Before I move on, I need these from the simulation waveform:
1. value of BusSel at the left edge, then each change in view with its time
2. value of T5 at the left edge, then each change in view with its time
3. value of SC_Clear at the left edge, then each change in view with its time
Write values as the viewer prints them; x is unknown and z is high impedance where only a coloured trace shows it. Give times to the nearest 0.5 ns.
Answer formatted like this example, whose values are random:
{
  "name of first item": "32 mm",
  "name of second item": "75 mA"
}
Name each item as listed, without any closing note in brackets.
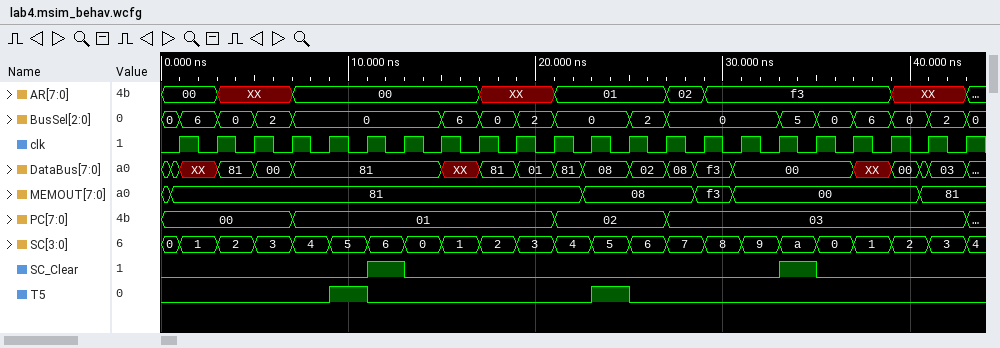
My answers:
{
  "value of BusSel at the left edge, then each change in view with its time": "0, 6 at 1 ns, 0 at 3 ns, 2 at 5 ns, 0 at 7 ns, 6 at 15 ns, 0 at 17 ns, 2 at 19 ns, 0 at 21 ns, 2 at 25 ns, 0 at 27 ns, 5 at 33 ns, 0 at 35 ns, 6 at 37 ns, 0 at 39 ns, 2 at 41 ns, 0 at 43 ns",
  "value of T5 at the left edge, then each change in view with its time": "0, 1 at 9 ns, 0 at 11 ns, 1 at 23 ns, 0 at 25 ns",
  "value of SC_Clear at the left edge, then each change in view with its time": "0, 1 at 11 ns, 0 at 13 ns, 1 at 33 ns, 0 at 35 ns"
}
